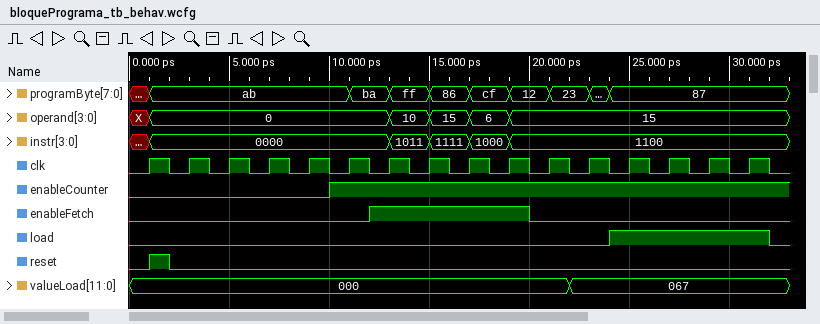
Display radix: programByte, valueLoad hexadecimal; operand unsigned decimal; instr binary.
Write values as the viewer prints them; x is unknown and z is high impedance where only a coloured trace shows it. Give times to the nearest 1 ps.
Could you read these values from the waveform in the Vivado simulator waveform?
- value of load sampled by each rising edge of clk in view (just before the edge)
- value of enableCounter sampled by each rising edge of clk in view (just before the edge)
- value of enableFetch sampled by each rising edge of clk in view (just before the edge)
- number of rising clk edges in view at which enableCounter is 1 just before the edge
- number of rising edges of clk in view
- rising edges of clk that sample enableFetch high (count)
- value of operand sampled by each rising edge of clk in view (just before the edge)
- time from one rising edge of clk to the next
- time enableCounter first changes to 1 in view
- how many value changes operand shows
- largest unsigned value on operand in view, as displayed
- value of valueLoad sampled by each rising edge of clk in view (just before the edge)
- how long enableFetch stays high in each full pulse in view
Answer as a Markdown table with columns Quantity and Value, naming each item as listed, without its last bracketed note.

| Quantity | Value |
|---|---|
| value of load sampled by each rising edge of clk in view | 0 0 0 0 0 0 0 0 0 0 0 0 1 1 1 1 |
| value of enableCounter sampled by each rising edge of clk in view | 0 0 0 0 0 1 1 1 1 1 1 1 1 1 1 1 |
| value of enableFetch sampled by each rising edge of clk in view | 0 0 0 0 0 0 1 1 1 1 0 0 0 0 0 0 |
| number of rising clk edges in view at which enableCounter is 1 just before the edge | 11 |
| number of rising edges of clk in view | 16 |
| rising edges of clk that sample enableFetch high | 4 |
| value of operand sampled by each rising edge of clk in view | X, 0, 0, 0, 0, 0, 0, 10, 15, 6, 15, 15, 15, 15, 15, 15 |
| time from one rising edge of clk to the next | 2 ps |
| time enableCounter first changes to 1 in view | 10 ps |
| how many value changes operand shows | 5 |
| largest unsigned value on operand in view, as displayed | 15 |
| value of valueLoad sampled by each rising edge of clk in view | 000, 000, 000, 000, 000, 000, 000, 000, 000, 000, 000, 067, 067, 067, 067, 067 |
| how long enableFetch stays high in each full pulse in view | 8 ps |
